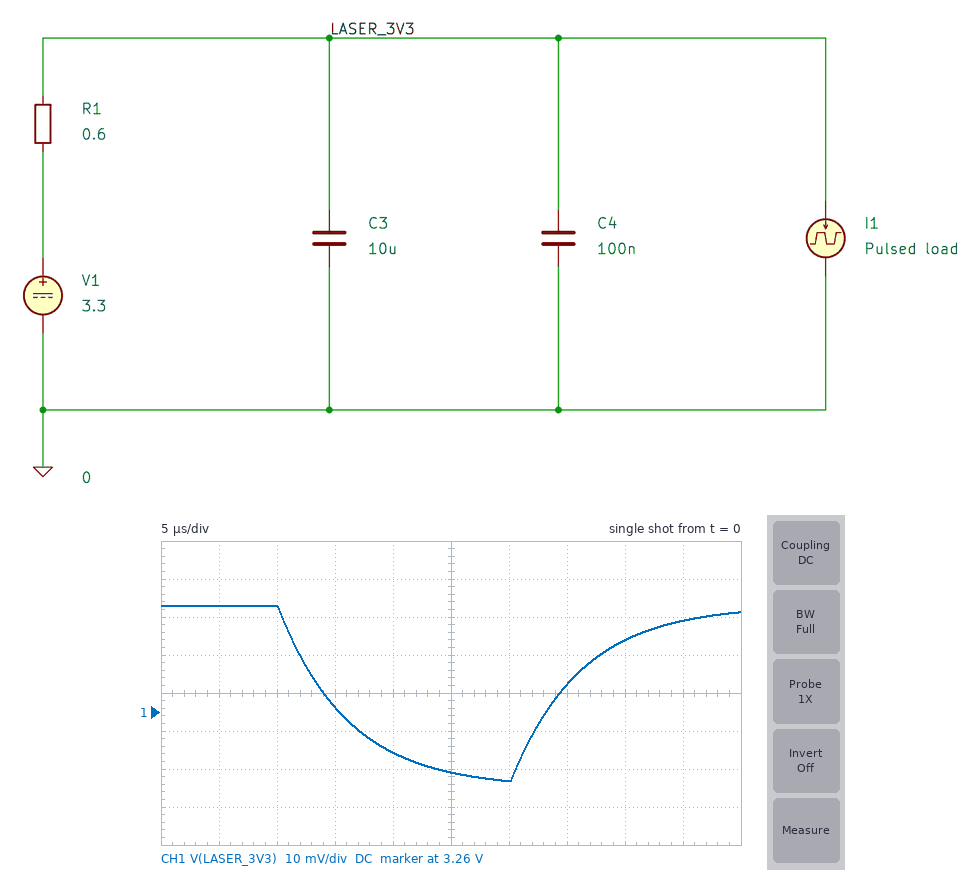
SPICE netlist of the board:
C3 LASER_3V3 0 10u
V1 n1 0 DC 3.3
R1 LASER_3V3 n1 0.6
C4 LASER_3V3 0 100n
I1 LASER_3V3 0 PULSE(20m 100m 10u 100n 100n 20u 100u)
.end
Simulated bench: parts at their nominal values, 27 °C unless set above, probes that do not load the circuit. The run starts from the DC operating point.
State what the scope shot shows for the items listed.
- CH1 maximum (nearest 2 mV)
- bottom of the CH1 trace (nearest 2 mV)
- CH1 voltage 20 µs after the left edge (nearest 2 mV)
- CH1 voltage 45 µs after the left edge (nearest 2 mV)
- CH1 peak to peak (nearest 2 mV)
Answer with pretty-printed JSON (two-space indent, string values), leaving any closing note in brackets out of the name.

{
  "CH1 maximum": "3.288 V",
  "bottom of the CH1 trace": "3.242 V",
  "CH1 voltage 20 µs after the left edge": "3.250 V",
  "CH1 voltage 45 µs after the left edge": "3.284 V",
  "CH1 peak to peak": "46 mV"
}
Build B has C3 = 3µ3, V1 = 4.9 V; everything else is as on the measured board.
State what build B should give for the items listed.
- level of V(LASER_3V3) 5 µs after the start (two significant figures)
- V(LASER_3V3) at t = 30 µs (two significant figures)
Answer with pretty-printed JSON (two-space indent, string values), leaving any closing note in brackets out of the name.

{
  "level of V(LASER_3V3) 5 µs after the start": "4.9 V",
  "V(LASER_3V3) at t = 30 µs": "4.8 V"
}
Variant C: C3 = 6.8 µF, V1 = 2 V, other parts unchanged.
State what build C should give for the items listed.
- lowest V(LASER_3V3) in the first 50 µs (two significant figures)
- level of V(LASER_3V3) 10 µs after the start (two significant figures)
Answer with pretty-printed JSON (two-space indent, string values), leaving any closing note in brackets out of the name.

{
  "lowest V(LASER_3V3) in the first 50 µs": "1.9 V",
  "level of V(LASER_3V3) 10 µs after the start": "2.0 V"
}
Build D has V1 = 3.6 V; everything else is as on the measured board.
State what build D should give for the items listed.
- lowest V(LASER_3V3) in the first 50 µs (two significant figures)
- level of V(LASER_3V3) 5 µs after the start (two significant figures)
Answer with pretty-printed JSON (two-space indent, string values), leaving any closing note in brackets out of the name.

{
  "lowest V(LASER_3V3) in the first 50 µs": "3.5 V",
  "level of V(LASER_3V3) 5 µs after the start": "3.6 V"
}
